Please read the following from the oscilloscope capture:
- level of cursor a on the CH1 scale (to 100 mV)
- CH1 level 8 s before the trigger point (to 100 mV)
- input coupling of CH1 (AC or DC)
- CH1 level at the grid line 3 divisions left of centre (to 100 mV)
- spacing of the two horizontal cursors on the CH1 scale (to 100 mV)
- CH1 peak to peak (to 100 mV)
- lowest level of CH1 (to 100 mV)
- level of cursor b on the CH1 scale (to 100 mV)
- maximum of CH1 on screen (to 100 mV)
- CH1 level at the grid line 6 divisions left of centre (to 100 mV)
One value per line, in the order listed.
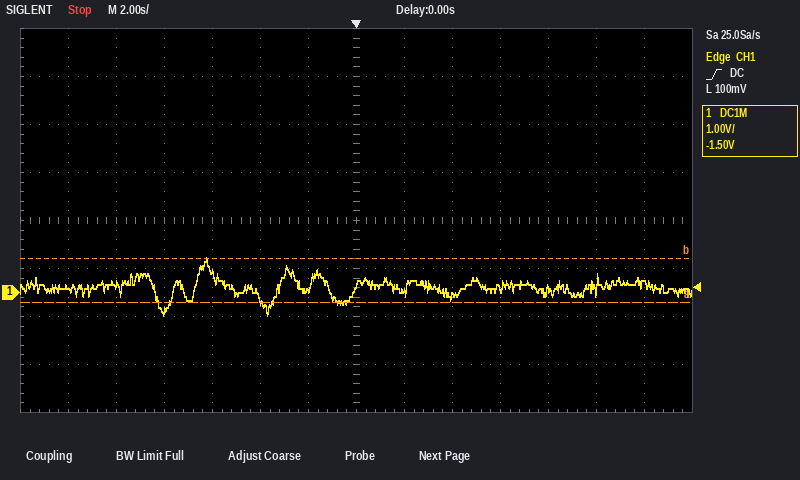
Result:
-200 mV
-400 mV
DC
400 mV
900 mV
1.2 V
-500 mV
700 mV
700 mV
100 mV
